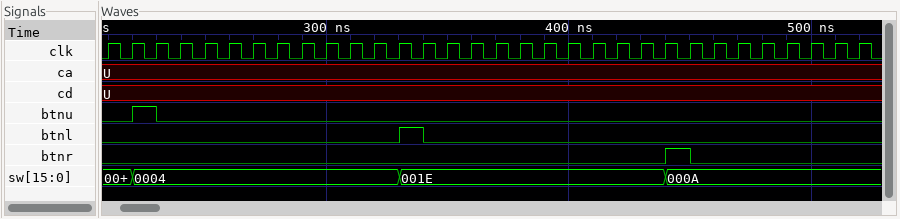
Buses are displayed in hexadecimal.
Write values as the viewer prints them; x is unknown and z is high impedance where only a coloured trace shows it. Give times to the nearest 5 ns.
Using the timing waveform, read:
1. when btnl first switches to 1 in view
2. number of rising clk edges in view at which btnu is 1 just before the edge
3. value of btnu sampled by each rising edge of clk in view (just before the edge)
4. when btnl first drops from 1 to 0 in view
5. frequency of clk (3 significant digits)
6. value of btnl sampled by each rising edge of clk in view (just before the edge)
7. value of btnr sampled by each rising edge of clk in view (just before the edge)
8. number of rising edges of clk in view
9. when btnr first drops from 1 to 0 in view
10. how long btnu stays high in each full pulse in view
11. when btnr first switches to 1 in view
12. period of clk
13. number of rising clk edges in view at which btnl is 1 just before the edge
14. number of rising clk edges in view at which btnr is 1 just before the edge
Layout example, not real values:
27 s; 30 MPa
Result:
330 ns; 1; 0 0 1 0 0 0 0 0 0 0 0 0 0 0 0 0 0 0 0 0 0 0 0 0 0 0 0 0 0 0 0 0; 340 ns; 100 MHz; 0 0 0 0 0 0 0 0 0 0 0 0 0 1 0 0 0 0 0 0 0 0 0 0 0 0 0 0 0 0 0 0; 0 0 0 0 0 0 0 0 0 0 0 0 0 0 0 0 0 0 0 0 0 0 0 0 1 0 0 0 0 0 0 0; 32; 450 ns; 10 ns; 440 ns; 10 ns; 1; 1
